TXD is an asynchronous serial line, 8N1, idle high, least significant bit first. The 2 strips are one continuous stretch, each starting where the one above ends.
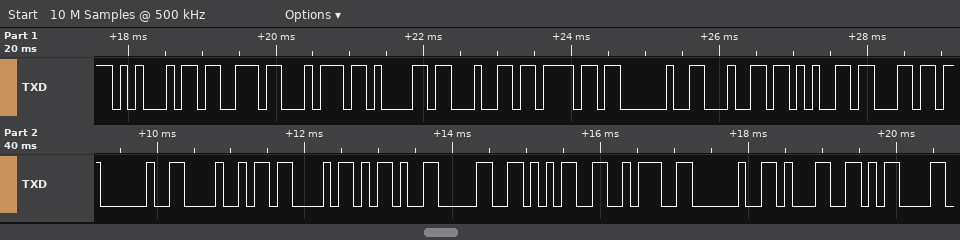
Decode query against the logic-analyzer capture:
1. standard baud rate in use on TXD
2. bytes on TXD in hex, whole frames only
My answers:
9600 baud
0x45 0x73 0x74 0x61 0x64 0x6F 0x20 0x64 0x65 0x6C 0x20 0x48 0x43 0x2D 0x30 0x35 0x3A 0x20 0x31 0x0D
